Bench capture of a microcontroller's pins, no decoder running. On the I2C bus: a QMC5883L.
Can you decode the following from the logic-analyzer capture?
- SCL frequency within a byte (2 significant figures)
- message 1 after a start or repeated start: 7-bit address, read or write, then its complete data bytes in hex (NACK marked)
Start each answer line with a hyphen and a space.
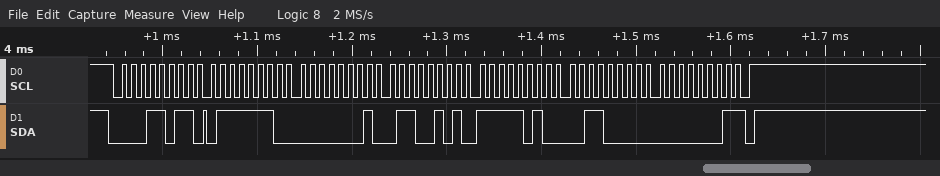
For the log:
- 100 kHz
- 0x0D read: 7E 01 65 FA 30 01 NACK
